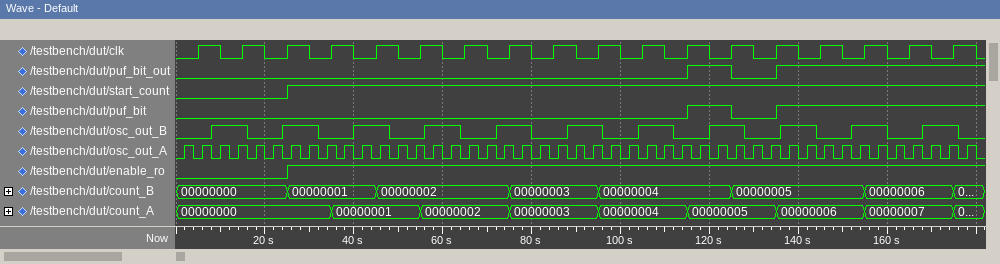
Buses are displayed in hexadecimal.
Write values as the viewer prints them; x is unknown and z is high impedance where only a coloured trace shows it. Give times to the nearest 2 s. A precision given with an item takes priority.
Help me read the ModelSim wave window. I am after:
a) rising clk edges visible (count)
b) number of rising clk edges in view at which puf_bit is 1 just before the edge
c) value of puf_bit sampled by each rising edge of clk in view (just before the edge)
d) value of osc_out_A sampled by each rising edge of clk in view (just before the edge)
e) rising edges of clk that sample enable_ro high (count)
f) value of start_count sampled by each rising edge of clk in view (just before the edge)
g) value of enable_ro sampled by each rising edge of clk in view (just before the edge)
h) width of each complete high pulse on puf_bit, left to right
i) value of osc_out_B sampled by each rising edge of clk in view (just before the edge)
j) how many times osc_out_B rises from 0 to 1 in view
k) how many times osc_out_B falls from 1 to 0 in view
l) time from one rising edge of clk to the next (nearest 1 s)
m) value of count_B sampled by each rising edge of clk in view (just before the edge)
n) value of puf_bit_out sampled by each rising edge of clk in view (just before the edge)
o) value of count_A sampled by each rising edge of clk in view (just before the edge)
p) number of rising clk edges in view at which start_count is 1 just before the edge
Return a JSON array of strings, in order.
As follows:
["18", "5", "0 0 0 0 0 0 0 0 0 0 0 0 1 0 1 1 1 1", "0 1 0 1 0 1 0 1 0 1 0 1 0 1 0 1 0 1", "15", "0 0 0 1 1 1 1 1 1 1 1 1 1 1 1 1 1 1", "0 0 0 1 1 1 1 1 1 1 1 1 1 1 1 1 1 1", "10 s", "0 1 1 0 1 0 0 1 0 1 1 0 1 0 0 1 0 1", "11", "11", "10 s", "00000000, 00000000, 00000000, 00000001, 00000001, 00000002, 00000002, 00000002, 00000003, 00000003, 00000004, 00000004, 00000004, 00000005, 00000005, 00000005, 00000006, 00000006", "0 0 0 0 0 0 0 0 0 0 0 0 1 0 1 1 1 1", "00000000, 00000000, 00000000, 00000000, 00000001, 00000001, 00000002, 00000002, 00000003, 00000003, 00000004, 00000004, 00000005, 00000005, 00000006, 00000006, 00000007, 00000007", "15"]
